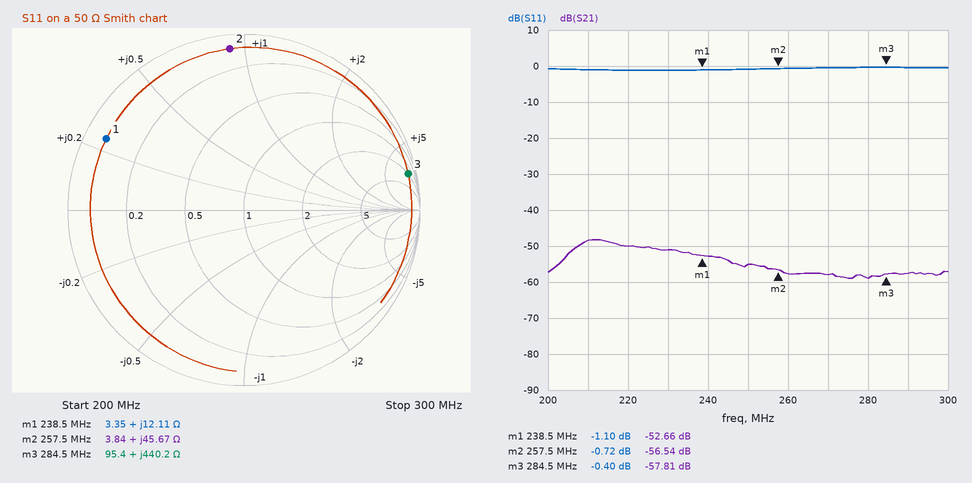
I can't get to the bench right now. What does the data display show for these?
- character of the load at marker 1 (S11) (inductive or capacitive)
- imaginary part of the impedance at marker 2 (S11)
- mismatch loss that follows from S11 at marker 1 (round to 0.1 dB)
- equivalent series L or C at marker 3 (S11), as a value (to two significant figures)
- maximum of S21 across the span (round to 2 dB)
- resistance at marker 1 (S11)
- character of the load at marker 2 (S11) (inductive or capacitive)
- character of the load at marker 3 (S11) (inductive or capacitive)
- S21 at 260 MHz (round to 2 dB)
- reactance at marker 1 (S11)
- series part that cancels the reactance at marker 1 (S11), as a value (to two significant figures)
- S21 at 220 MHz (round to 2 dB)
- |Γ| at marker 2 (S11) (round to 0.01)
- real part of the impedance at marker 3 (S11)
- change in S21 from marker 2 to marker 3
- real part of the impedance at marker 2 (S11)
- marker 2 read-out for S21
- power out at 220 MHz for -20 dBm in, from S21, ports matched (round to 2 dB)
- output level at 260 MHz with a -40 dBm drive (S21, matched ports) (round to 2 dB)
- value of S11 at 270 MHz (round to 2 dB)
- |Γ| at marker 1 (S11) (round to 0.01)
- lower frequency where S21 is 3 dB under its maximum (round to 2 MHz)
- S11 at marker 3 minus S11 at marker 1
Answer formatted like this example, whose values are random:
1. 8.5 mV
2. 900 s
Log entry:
1. inductive
2. +45.67 Ω
3. 6.5 dB
4. 250 nH
5. -48 dB
6. 3.35 Ω
7. inductive
8. inductive
9. -58 dB
10. +12.11 Ω
11. 55 pF
12. -50 dB
13. 0.92
14. 95.4 Ω
15. -1.27 dB
16. 3.84 Ω
17. -56.54 dB
18. -70 dBm
19. -98 dBm
20. 0 dB
21. 0.88
22. 206 MHz
23. 0.70 dB
